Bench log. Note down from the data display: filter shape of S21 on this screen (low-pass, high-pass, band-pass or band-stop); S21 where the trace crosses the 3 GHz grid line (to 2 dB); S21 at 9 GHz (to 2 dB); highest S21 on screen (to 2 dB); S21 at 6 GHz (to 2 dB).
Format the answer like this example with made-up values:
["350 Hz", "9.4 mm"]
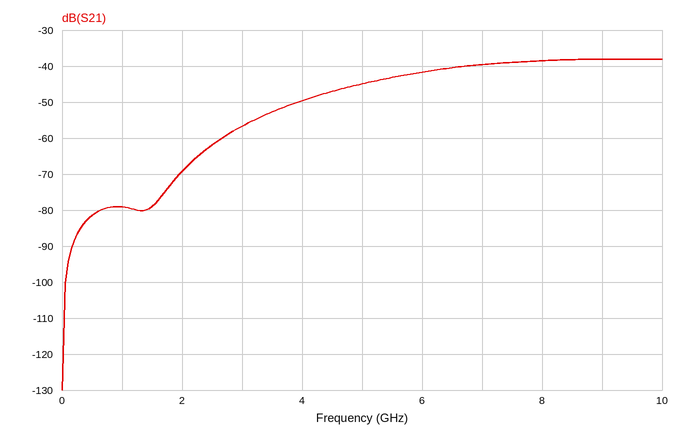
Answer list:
["high-pass", "-56 dB", "-38 dB", "-38 dB", "-42 dB"]
